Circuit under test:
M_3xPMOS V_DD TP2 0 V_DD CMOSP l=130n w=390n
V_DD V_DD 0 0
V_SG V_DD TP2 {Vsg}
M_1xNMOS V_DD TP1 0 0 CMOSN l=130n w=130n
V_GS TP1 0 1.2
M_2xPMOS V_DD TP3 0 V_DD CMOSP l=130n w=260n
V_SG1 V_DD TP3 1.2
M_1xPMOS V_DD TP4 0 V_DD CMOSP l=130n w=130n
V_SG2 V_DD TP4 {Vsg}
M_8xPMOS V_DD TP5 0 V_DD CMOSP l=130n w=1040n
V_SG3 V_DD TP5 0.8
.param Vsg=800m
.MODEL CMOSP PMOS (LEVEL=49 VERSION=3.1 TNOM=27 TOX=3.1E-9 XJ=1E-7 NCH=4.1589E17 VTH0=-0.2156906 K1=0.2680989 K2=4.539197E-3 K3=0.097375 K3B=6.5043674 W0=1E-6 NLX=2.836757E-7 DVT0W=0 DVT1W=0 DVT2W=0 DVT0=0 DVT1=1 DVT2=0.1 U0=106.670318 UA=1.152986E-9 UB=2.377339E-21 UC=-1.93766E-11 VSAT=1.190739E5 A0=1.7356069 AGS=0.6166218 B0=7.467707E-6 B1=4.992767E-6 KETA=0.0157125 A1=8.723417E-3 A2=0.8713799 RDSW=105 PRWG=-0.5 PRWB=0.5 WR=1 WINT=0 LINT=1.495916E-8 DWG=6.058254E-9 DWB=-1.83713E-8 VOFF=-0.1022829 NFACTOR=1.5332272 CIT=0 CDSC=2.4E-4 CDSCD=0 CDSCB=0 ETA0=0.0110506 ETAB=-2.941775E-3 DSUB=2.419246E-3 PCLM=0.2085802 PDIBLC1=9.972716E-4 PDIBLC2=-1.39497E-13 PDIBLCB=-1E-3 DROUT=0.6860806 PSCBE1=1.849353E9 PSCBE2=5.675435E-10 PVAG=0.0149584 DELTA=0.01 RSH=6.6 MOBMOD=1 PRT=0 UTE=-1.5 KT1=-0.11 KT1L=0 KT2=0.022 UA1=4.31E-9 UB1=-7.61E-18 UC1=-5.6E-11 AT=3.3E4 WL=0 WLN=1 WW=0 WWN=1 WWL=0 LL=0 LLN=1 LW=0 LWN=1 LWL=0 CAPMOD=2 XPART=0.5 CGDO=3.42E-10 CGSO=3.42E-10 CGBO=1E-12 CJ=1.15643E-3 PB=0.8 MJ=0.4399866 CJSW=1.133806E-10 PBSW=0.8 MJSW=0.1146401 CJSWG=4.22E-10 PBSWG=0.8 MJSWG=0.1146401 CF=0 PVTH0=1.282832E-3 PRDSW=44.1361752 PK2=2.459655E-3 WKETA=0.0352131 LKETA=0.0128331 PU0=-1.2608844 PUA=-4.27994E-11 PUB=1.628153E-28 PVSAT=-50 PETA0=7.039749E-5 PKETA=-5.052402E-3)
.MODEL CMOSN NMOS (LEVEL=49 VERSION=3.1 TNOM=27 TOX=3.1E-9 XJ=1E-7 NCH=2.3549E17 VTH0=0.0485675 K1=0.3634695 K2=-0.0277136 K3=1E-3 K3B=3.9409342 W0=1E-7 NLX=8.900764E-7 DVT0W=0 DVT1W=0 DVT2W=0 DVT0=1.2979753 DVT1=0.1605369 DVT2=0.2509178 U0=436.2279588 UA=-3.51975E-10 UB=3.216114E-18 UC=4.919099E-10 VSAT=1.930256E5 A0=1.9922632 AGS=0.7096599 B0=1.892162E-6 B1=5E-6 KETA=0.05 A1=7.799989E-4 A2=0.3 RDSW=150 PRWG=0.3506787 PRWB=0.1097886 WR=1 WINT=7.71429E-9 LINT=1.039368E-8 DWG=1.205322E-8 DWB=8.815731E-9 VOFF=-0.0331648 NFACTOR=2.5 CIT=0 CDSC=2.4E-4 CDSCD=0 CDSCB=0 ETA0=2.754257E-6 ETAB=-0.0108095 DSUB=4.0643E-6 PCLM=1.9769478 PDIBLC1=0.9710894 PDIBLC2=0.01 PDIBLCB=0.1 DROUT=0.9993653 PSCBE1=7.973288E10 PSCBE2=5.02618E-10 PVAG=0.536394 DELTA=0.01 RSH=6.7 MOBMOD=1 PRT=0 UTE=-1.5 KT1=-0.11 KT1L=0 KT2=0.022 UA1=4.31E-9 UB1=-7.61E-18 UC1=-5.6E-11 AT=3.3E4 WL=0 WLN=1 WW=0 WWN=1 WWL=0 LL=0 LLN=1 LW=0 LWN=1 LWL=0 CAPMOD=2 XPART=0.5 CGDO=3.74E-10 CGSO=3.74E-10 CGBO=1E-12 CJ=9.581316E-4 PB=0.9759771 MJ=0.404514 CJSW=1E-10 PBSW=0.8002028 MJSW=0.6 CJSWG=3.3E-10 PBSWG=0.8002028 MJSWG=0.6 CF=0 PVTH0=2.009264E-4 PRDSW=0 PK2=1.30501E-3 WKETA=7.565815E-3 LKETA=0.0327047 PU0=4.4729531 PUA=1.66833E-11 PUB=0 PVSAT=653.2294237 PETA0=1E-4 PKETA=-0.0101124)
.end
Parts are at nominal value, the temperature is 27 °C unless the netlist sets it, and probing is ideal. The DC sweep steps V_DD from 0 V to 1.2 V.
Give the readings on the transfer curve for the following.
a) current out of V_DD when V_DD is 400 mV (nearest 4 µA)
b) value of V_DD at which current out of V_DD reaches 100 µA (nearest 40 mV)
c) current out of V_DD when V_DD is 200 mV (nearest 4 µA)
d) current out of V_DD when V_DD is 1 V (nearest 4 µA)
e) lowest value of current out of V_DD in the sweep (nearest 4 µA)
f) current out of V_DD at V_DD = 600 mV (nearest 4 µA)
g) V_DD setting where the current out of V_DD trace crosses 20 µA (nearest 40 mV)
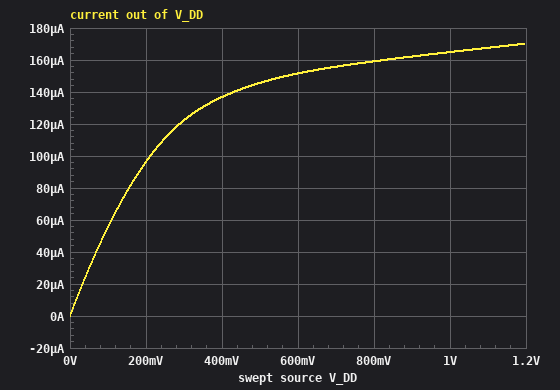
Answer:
136 µA
200 mV
96 µA
164 µA
0 A
152 µA
40 mV
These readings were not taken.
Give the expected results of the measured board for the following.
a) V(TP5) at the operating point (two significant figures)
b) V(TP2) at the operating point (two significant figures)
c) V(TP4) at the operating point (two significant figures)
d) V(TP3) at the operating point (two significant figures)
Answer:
-800 mV
-800 mV
-800 mV
-1.2 V
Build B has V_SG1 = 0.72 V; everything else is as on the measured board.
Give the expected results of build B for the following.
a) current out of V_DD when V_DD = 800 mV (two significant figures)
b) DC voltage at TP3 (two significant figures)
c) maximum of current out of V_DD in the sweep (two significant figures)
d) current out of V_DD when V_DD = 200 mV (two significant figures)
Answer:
130 µA
-720 mV
140 µA
85 µA
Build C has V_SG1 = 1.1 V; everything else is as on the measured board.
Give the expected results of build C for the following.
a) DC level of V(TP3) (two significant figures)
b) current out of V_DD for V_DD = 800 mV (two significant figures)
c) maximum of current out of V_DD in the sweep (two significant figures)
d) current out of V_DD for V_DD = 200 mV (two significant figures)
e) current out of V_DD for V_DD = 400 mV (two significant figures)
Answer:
-1.1 V
150 µA
160 µA
94 µA
130 µA
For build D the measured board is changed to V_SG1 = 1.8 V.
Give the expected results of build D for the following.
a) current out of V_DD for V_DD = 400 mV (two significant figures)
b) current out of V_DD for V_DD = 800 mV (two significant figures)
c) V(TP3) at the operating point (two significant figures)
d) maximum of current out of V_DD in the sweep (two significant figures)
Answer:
170 µA
220 µA
-1.8 V
240 µA
